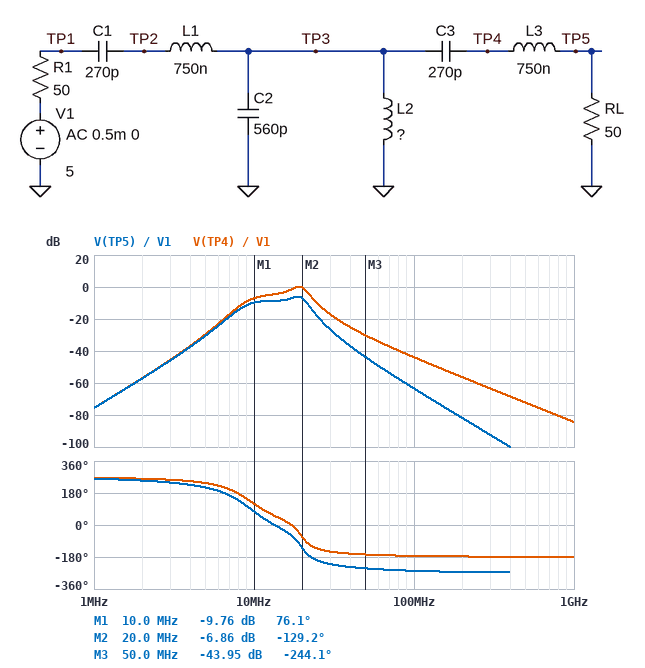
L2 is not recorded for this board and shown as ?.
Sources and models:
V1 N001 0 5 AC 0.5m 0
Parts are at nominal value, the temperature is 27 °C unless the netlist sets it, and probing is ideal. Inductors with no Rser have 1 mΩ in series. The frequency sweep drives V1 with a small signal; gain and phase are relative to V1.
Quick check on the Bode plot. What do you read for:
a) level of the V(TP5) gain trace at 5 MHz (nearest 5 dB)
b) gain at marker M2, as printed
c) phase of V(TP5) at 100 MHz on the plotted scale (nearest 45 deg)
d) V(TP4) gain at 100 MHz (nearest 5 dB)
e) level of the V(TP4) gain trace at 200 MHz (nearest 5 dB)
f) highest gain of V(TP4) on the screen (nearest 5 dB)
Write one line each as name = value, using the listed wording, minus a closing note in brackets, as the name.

level of the V(TP5) gain trace at 5 MHz = -30 dB
gain at marker M2, as printed = -6.86 dB
phase of V(TP5) at 100 MHz on the plotted scale = -270 deg
V(TP4) gain at 100 MHz = -45 dB
level of the V(TP4) gain trace at 200 MHz = -55 dB
highest gain of V(TP4) on the screen = 0 dB
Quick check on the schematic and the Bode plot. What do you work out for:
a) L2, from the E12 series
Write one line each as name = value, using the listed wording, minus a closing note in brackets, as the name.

L2, from the E12 series = 180 nH
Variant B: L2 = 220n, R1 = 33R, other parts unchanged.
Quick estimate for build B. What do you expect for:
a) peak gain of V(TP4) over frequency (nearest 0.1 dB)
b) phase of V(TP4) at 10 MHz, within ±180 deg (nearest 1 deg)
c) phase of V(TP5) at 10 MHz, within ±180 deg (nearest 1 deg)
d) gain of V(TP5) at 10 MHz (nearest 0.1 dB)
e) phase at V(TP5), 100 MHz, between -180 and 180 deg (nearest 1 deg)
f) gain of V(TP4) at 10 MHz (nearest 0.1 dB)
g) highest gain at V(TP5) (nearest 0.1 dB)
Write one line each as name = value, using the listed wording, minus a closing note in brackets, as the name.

peak gain of V(TP4) over frequency = 1.7 dB
phase of V(TP4) at 10 MHz, within ±180 deg = 103 deg
phase of V(TP5) at 10 MHz, within ±180 deg = 60 deg
gain of V(TP5) at 10 MHz = -5.3 dB
phase at V(TP5), 100 MHz, between -180 and 180 deg = 100 deg
gain of V(TP4) at 10 MHz = -2.6 dB
highest gain at V(TP5) = -4.2 dB
